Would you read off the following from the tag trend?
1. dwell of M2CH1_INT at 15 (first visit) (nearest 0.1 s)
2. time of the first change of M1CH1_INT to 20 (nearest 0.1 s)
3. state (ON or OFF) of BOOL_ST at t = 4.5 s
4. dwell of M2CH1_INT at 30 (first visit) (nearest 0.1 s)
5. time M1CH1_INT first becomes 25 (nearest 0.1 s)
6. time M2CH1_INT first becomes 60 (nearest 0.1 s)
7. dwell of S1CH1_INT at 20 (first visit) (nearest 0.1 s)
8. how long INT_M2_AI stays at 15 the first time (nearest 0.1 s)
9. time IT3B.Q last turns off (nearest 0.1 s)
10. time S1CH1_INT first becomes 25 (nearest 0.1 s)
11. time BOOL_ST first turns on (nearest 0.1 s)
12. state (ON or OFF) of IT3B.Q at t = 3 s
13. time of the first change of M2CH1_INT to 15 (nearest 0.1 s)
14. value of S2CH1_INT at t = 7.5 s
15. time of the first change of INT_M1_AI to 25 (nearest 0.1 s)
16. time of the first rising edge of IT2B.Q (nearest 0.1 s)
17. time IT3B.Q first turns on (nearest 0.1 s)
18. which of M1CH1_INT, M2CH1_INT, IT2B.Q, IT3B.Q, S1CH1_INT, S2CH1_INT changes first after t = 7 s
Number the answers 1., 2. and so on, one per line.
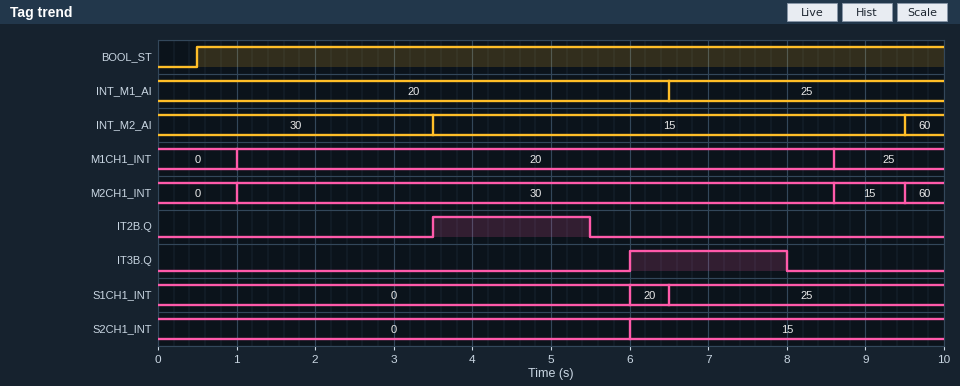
1. 0.9 s
2. 1.0 s
3. ON
4. 7.6 s
5. 8.6 s
6. 9.5 s
7. 0.5 s
8. 6.0 s
9. 8.0 s
10. 6.5 s
11. 0.5 s
12. OFF
13. 8.6 s
14. 15
15. 6.5 s
16. 3.5 s
17. 6.0 s
18. IT3B.Q
